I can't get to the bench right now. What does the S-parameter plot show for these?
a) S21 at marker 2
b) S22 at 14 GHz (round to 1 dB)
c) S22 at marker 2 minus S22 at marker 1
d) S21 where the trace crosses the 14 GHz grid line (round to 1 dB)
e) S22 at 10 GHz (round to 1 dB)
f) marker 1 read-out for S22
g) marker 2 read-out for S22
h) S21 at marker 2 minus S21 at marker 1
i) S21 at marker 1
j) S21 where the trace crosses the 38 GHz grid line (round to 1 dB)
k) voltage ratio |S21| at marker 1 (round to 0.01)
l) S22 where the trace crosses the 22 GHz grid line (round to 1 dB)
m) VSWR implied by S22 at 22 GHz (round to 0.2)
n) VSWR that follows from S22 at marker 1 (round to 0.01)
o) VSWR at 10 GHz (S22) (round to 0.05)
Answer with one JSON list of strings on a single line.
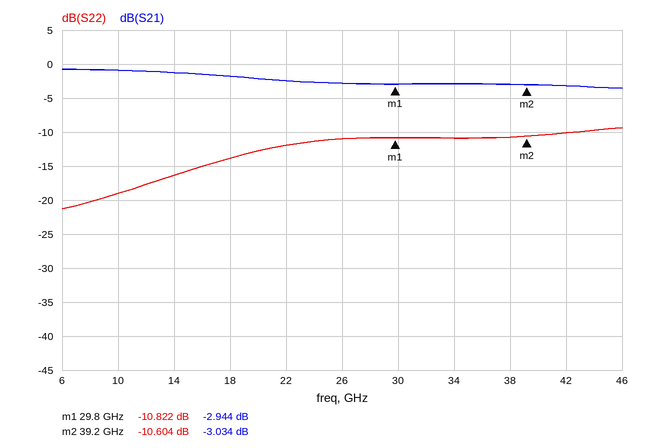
["-3.034 dB", "-16 dB", "0.218 dB", "-1 dB", "-19 dB", "-10.822 dB", "-10.604 dB", "-0.090 dB", "-2.944 dB", "-3 dB", "0.71", "-12 dB", "1.6", "1.81", "1.25"]
